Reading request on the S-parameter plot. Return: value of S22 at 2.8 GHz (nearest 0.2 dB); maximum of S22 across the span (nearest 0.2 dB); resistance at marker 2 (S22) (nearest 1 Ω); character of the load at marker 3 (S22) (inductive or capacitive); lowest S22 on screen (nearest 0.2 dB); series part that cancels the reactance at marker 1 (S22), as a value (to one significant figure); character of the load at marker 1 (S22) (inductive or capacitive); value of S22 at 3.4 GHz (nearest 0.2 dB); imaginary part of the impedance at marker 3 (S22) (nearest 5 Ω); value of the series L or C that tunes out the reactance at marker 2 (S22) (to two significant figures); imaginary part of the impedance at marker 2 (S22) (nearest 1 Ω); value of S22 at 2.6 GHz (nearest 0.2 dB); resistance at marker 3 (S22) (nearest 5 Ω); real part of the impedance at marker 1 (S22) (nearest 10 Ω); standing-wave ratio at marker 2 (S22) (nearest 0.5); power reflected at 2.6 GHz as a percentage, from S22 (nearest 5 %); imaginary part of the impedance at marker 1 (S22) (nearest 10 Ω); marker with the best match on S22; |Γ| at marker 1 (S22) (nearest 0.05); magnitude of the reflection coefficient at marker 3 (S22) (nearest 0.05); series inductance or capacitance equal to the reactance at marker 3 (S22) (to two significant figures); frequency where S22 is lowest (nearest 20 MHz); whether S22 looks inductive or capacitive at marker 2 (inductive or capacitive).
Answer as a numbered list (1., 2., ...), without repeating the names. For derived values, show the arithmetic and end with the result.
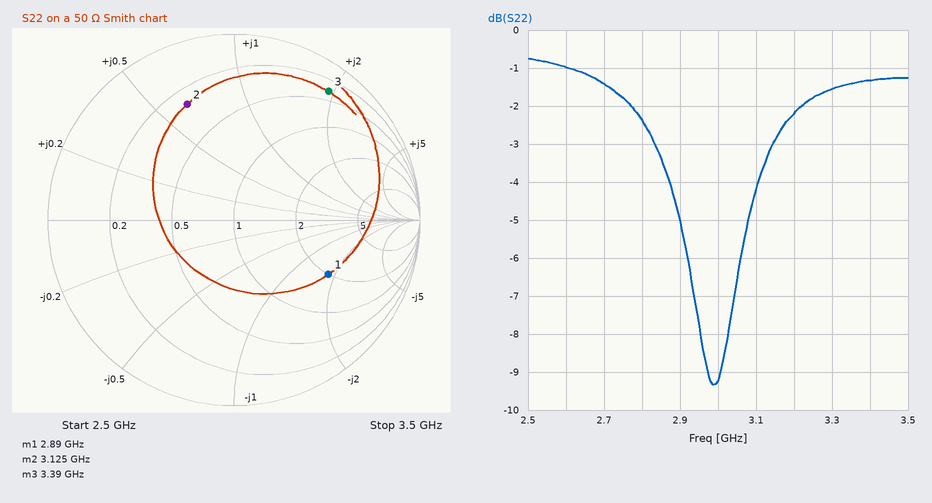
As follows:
1. -2.4 dB
2. -0.8 dB
3. 14 Ω
4. inductive
5. -9.4 dB
6. L = 90 Ω/(2π × 2.89 GHz) ≈ 5 nH
7. capacitive
8. -1.4 dB
9. +95 Ω
10. C = 1/(2π × 3.125 GHz × 32 Ω) ≈ 1.6 pF
11. +32 Ω
12. -1.0 dB
13. 20 Ω
14. 100 Ω
15. 5.0
16. 10^(-1/10) ≈ 79.4 %, so 80 % to the nearest 5 %
17. -90 Ω
18. marker 1
19. 0.60
20. 0.85
21. L = 95 Ω/(2π × 3.39 GHz) ≈ 4.5 nH
22. 2.98 GHz
23. inductive
